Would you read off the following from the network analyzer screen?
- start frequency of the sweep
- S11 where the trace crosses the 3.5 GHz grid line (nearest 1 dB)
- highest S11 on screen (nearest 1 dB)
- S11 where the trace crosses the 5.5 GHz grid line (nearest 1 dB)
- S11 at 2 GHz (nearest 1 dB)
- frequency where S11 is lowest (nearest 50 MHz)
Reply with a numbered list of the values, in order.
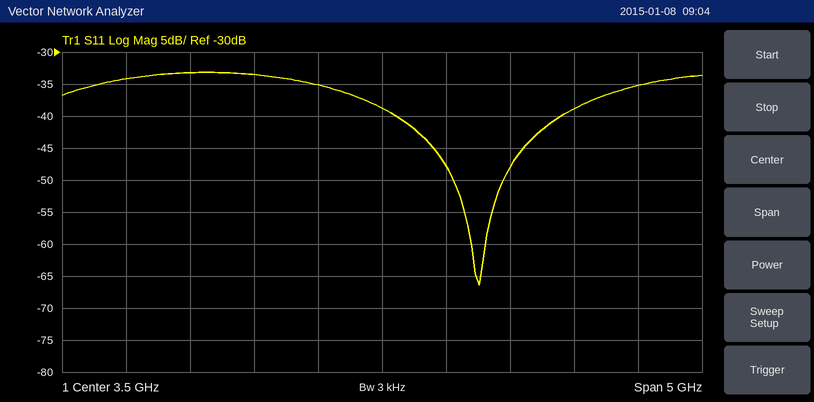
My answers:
1. 1 GHz
2. -39 dB
3. -33 dB
4. -35 dB
5. -33 dB
6. 4.25 GHz
